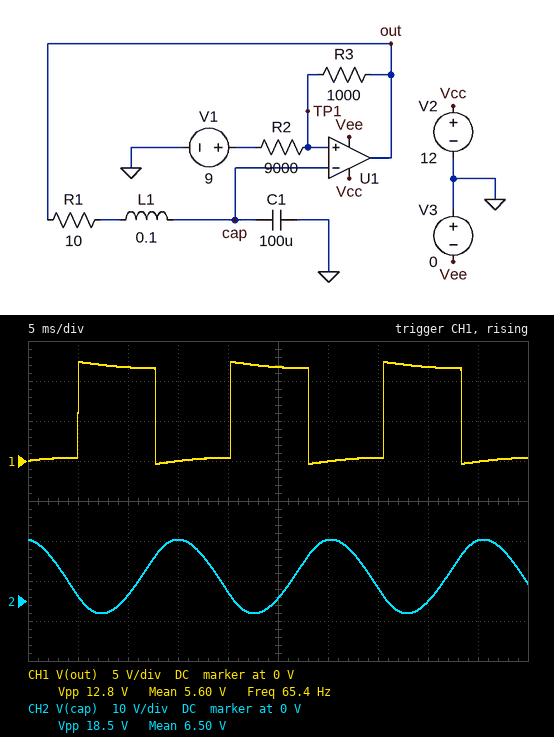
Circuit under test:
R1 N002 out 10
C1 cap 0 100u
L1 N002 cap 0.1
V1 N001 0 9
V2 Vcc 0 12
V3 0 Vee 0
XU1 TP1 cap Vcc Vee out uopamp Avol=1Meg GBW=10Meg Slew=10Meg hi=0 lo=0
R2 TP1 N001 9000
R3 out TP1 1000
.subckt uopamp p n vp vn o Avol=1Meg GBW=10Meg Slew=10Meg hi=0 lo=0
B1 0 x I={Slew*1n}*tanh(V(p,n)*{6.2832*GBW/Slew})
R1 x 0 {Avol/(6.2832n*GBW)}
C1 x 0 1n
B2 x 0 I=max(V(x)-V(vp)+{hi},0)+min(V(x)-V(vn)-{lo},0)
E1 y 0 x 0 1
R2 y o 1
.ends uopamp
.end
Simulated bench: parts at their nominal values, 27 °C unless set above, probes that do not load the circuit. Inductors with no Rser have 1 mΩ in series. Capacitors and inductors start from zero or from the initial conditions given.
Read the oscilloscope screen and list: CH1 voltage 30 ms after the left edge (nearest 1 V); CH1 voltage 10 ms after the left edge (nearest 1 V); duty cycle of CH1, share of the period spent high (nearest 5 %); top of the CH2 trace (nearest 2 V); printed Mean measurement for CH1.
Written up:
0 V
12 V
50 %
16 V
5.60 V
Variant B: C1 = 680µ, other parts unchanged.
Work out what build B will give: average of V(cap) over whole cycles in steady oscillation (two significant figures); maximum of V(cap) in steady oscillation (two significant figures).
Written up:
6.2 V
12 V
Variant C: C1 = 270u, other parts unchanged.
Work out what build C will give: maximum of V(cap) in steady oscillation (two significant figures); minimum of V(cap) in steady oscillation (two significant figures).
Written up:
13 V
-1.0 V
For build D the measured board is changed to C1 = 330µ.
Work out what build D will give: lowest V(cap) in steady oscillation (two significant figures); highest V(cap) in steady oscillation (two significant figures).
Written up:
-670 mV
13 V
